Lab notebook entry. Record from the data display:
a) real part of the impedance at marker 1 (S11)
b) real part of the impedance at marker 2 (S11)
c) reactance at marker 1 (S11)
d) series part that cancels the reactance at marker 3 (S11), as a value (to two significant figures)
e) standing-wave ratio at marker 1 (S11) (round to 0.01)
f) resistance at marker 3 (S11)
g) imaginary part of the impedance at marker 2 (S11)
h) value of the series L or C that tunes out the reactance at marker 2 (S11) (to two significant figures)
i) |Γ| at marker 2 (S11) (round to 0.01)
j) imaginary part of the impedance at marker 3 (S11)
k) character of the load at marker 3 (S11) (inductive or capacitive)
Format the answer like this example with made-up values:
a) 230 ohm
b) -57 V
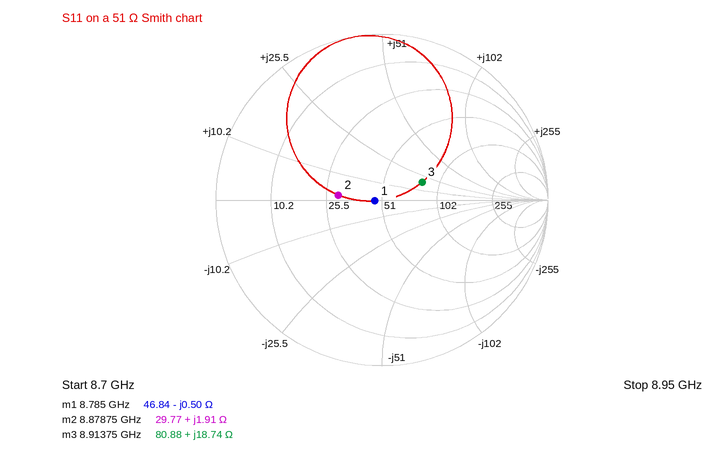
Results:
a) 46.84 Ω
b) 29.77 Ω
c) -0.50 Ω
d) 950 fF
e) 1.09
f) 80.88 Ω
g) +1.91 Ω
h) 9.4 pF
i) 0.26
j) +18.74 Ω
k) inductive
